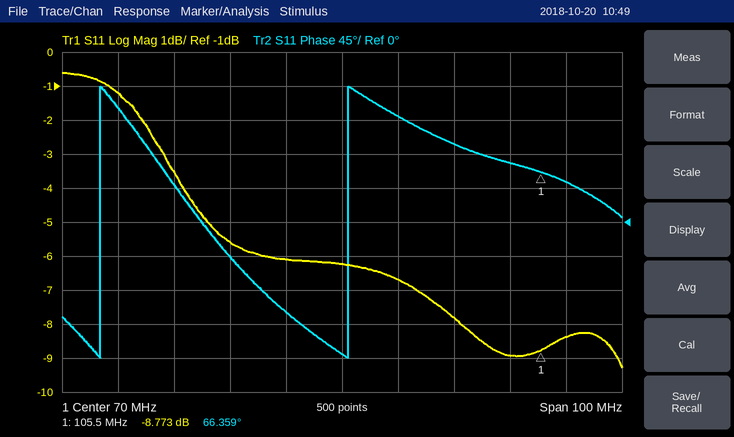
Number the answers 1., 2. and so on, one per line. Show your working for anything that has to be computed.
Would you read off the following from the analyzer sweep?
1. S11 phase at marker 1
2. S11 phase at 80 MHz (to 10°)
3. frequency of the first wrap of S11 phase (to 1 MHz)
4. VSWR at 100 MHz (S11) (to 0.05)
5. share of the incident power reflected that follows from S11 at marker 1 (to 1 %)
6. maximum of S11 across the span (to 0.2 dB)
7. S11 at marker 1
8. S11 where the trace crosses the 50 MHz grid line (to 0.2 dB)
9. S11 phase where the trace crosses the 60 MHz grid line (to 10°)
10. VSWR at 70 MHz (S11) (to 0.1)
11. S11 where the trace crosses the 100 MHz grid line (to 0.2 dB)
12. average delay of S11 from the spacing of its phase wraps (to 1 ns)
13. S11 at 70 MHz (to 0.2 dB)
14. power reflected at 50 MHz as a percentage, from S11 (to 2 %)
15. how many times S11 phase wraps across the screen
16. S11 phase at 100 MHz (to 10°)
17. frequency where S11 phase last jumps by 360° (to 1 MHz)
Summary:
1. 66.359°
2. 140°
3. 27 MHz
4. |Γ| = 10^(-9/20) = 0.3548; VSWR = (1 + 0.3548)/(1 − 0.3548) ≈ 2.10
5. 10^(-8.773/10) ≈ 13 %
6. -0.6 dB
7. -8.773 dB
8. -5.6 dB
9. -120°
10. |Γ| = 10^(-6.2/20) = 0.4898; VSWR = (1 + 0.4898)/(1 − 0.4898) ≈ 2.9
11. -9.0 dB
12. 1 cycle / (71 MHz − 27 MHz) ≈ 23 ns
13. -6.2 dB
14. 10^(-5.6/10) ≈ 28 %
15. 2
16. 80°
17. 71 MHz
